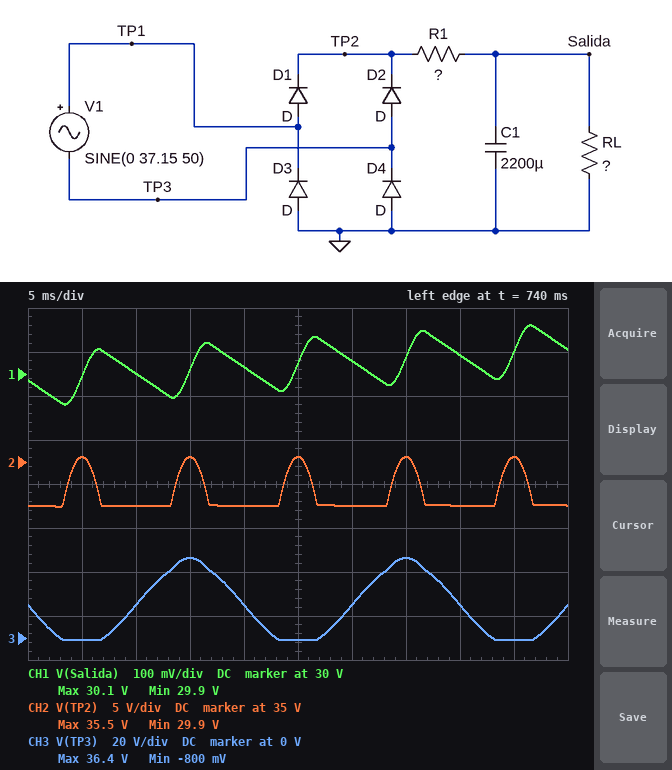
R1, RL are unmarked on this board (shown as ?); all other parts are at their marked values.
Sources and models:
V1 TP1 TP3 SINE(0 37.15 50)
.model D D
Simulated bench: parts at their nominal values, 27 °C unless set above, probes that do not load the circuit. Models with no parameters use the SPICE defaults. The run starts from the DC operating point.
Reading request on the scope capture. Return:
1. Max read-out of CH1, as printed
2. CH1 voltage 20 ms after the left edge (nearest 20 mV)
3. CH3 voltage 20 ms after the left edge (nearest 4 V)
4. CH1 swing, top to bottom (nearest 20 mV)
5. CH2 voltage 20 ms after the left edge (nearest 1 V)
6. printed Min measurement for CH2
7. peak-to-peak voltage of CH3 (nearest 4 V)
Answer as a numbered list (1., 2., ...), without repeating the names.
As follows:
1. 30.1 V
2. 30.02 V
3. 16 V
4. 180 mV
5. 30 V
6. 29.9 V
7. 36 V
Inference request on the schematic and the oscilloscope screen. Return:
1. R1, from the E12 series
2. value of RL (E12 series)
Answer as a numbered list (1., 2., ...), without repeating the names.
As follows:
1. 33 Ω
2. 820 Ω
